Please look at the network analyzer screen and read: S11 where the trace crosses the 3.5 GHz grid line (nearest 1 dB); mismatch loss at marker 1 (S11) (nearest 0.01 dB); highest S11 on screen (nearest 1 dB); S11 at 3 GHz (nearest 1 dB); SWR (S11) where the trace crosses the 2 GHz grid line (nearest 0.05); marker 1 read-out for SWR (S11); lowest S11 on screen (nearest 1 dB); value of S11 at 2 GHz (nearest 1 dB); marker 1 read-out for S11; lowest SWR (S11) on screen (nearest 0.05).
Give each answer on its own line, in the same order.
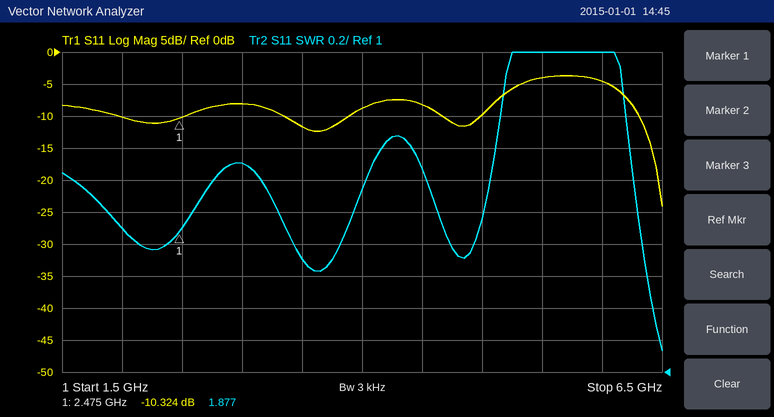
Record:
-12 dB
0.42 dB
-4 dB
-8 dB
1.90
1.877
-24 dB
-10 dB
-10.324 dB
1.15
